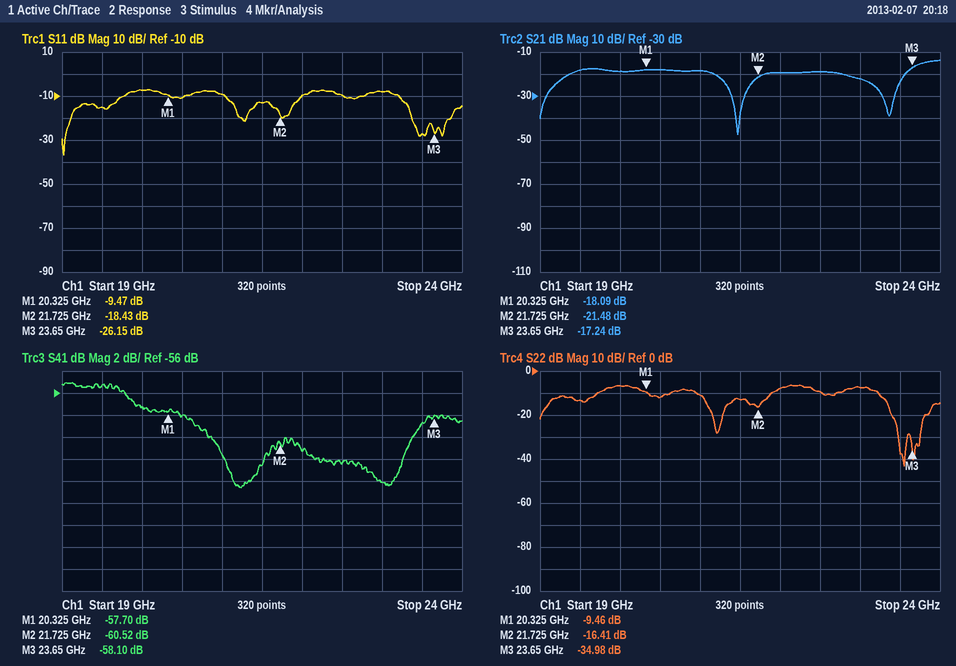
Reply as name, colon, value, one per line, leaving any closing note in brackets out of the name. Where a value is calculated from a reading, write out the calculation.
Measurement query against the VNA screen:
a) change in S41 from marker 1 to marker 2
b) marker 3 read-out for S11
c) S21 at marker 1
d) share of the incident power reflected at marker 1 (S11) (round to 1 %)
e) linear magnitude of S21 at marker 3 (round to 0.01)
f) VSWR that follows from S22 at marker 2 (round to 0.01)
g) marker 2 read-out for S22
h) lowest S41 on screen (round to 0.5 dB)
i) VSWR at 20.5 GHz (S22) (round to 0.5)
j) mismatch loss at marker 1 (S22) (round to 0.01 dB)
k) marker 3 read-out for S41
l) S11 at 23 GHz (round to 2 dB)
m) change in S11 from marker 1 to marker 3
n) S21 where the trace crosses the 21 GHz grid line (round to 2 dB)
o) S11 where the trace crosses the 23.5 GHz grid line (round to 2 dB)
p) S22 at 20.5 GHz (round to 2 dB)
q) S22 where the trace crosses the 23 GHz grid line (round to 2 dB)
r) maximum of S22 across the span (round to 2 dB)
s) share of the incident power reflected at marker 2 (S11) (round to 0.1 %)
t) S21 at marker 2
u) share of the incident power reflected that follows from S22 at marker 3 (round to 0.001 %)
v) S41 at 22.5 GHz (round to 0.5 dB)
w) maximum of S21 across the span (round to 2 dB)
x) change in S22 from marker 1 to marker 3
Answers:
change in S41 from marker 1 to marker 2: -60.52 − (-57.7) = -2.82 dB
marker 3 read-out for S11: -26.15 dB
S21 at marker 1: -18.09 dB
share of the incident power reflected at marker 1 (S11): 10^(-9.47/10) ≈ 11 %
linear magnitude of S21 at marker 3: 10^(-17.24/20) ≈ 0.14
VSWR that follows from S22 at marker 2: (1 + 0.1512)/(1 − 0.1512) ≈ 1.36
marker 2 read-out for S22: -16.41 dB
lowest S41 on screen: -64.5 dB
VSWR at 20.5 GHz (S22): |Γ| = 10^(-12/20) = 0.2512; VSWR = (1 + 0.2512)/(1 − 0.2512) ≈ 1.67, so 1.5 to the nearest 0.5
mismatch loss at marker 1 (S22): −10 log10(1 − 10^(-9.46/10)) ≈ 0.52 dB
marker 3 read-out for S41: -58.10 dB
S11 at 23 GHz: -8 dB
change in S11 from marker 1 to marker 3: -26.15 − (-9.47) = -16.68 dB
S21 where the trace crosses the 21 GHz grid line: -18 dB
S11 where the trace crosses the 23.5 GHz grid line: -28 dB
S22 at 20.5 GHz: -12 dB
S22 where the trace crosses the 23 GHz grid line: -8 dB
maximum of S22 across the span: -6 dB
share of the incident power reflected at marker 2 (S11): 10^(-18.43/10) ≈ 1.4 %
S21 at marker 2: -21.48 dB
share of the incident power reflected that follows from S22 at marker 3: 10^(-34.98/10) ≈ 0.032 %
S41 at 22.5 GHz: -62.5 dB
maximum of S21 across the span: -14 dB
change in S22 from marker 1 to marker 3: -34.98 − (-9.46) = -25.52 dB
